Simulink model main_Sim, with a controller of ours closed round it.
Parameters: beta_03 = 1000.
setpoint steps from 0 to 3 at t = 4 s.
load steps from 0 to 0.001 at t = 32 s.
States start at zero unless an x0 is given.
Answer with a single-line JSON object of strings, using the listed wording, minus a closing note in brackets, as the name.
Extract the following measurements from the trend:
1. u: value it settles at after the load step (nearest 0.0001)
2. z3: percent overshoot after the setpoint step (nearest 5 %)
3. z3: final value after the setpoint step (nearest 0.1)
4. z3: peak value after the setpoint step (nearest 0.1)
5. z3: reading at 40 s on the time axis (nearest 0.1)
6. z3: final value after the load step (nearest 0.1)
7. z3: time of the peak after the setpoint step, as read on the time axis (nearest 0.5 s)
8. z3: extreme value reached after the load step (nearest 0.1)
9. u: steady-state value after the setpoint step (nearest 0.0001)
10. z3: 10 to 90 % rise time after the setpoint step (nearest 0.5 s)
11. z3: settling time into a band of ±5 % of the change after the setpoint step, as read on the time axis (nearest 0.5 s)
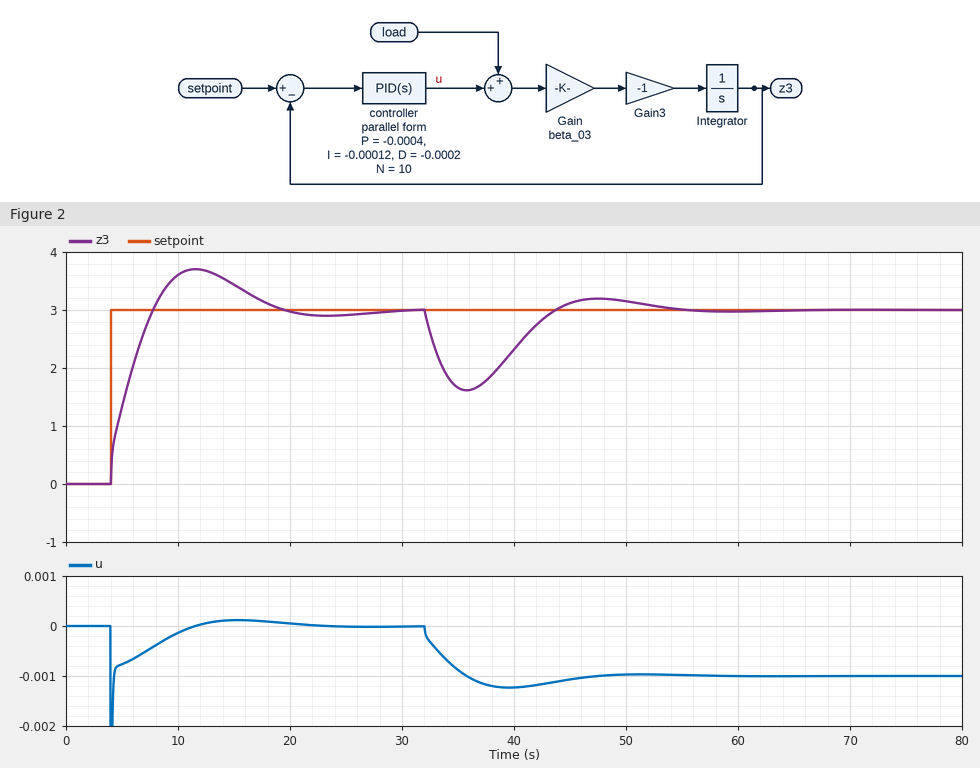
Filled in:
{"u: value it settles at after the load step": "-0.0010", "z3: percent overshoot after the setpoint step": "25 %", "z3: final value after the setpoint step": "3.0", "z3: peak value after the setpoint step": "3.7", "z3: reading at 40 s on the time axis": "2.3", "z3: final value after the load step": "3.0", "z3: time of the peak after the setpoint step, as read on the time axis": "11.5 s", "z3: extreme value reached after the load step": "1.6", "u: steady-state value after the setpoint step": "0.0000", "z3: 10 to 90 % rise time after the setpoint step": "3.0 s", "z3: settling time into a band of ±5 % of the change after the setpoint step, as read on the time axis": "17.5 s"}
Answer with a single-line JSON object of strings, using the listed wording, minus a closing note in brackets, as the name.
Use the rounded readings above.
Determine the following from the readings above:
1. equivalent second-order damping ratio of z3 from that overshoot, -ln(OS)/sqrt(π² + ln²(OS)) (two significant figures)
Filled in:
{"equivalent second-order damping ratio of z3 from that overshoot, -ln(OS)/sqrt(π² + ln²(OS))": "0.40"}
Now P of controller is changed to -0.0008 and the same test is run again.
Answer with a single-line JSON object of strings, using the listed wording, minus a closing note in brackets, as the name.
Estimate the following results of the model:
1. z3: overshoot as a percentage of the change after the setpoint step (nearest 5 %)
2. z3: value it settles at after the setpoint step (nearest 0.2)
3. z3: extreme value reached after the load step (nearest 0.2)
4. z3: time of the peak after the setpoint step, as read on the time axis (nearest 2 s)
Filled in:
{"z3: overshoot as a percentage of the change after the setpoint step": "10 %", "z3: value it settles at after the setpoint step": "3.0", "z3: extreme value reached after the load step": "2.0", "z3: time of the peak after the setpoint step, as read on the time axis": "10 s"}
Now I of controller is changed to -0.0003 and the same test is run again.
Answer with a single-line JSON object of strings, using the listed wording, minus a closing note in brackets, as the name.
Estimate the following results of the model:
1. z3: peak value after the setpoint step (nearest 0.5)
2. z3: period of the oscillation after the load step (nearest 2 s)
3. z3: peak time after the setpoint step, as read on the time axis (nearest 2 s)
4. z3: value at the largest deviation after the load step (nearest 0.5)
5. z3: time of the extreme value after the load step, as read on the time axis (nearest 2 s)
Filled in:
{"z3: peak value after the setpoint step": "4.0", "z3: period of the oscillation after the load step": "14 s", "z3: peak time after the setpoint step, as read on the time axis": "10 s", "z3: value at the largest deviation after the load step": "2.0", "z3: time of the extreme value after the load step, as read on the time axis": "34 s"}
